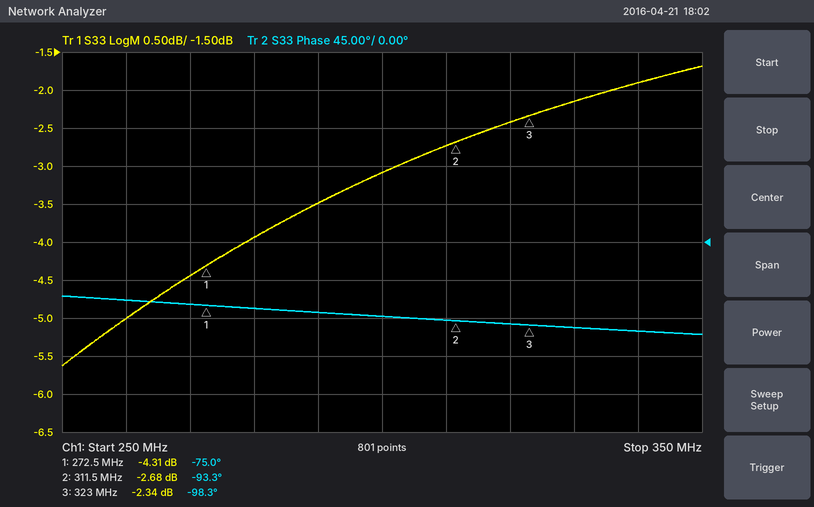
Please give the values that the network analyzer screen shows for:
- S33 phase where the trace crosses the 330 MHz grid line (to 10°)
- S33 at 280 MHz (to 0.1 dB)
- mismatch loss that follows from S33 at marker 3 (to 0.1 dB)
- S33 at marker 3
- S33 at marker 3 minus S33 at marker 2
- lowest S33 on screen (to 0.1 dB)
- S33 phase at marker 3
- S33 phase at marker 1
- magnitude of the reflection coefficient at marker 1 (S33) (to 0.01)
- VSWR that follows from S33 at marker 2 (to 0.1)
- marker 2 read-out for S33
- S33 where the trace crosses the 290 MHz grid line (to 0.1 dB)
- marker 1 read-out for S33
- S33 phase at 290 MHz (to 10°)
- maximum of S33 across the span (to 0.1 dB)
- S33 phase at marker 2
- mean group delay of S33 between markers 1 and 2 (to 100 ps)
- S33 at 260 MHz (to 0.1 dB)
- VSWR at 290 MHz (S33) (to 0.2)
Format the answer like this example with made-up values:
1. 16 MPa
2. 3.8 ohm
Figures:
1. -100°
2. -3.9 dB
3. 3.8 dB
4. -2.34 dB
5. 0.34 dB
6. -5.6 dB
7. -98.3°
8. -75.0°
9. 0.61
10. 6.5
11. -2.68 dB
12. -3.5 dB
13. -4.31 dB
14. -80°
15. -1.7 dB
16. -93.3°
17. 1.3 ns
18. -5.0 dB
19. 5.0
